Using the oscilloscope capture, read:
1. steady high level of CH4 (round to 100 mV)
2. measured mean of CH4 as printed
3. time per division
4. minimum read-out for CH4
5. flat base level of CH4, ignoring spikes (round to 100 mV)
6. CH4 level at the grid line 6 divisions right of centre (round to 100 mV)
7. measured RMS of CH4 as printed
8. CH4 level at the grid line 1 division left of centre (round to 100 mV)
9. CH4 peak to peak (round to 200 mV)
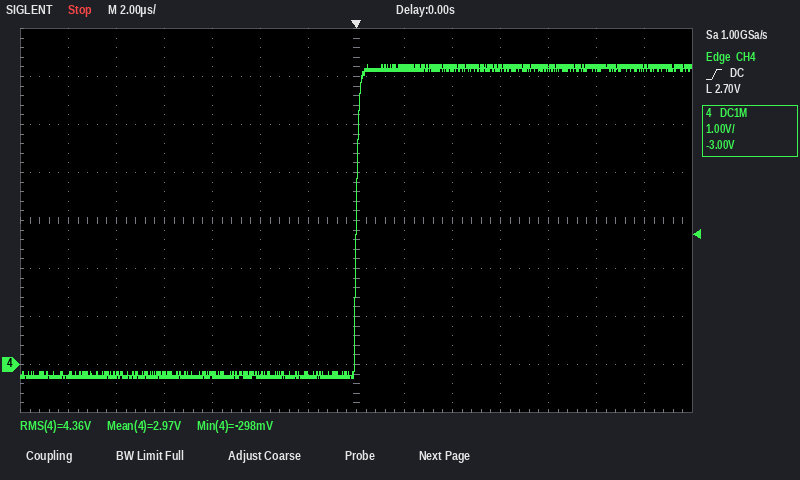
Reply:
6.2 V
2.97 V
2 µs
-298 mV
-200 mV
6.2 V
4.36 V
-200 mV
6.6 V
